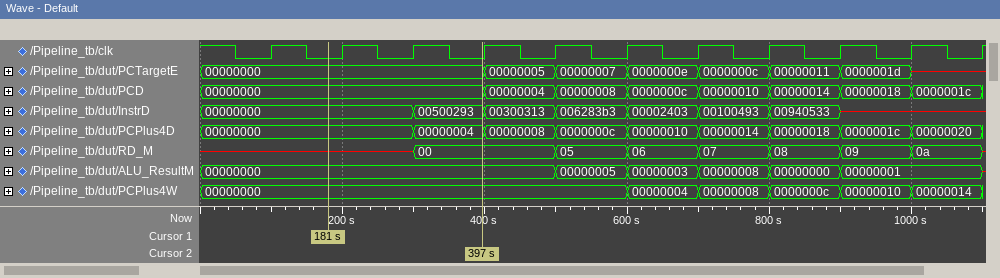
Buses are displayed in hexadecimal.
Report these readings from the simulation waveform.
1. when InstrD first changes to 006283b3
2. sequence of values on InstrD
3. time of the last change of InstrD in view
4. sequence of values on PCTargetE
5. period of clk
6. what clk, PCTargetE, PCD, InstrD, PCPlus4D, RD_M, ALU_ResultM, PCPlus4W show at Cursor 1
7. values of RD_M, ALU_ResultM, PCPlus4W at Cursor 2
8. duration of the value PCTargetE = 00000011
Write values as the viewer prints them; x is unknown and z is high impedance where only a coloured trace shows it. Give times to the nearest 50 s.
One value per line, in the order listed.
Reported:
500 s
00000000, 00500293, 00300313, 006283b3, 00002403, 00100493, 00940533, x
900 s
00000000, 00000005, 00000007, 0000000e, 0000000c, 00000011, 0000001d, x
100 s
clk=0, PCTargetE=00000000, PCD=00000000, InstrD=00000000, PCPlus4D=00000000, RD_M=x, ALU_ResultM=00000000, PCPlus4W=00000000
RD_M=00, ALU_ResultM=00000000, PCPlus4W=00000000
100 s
